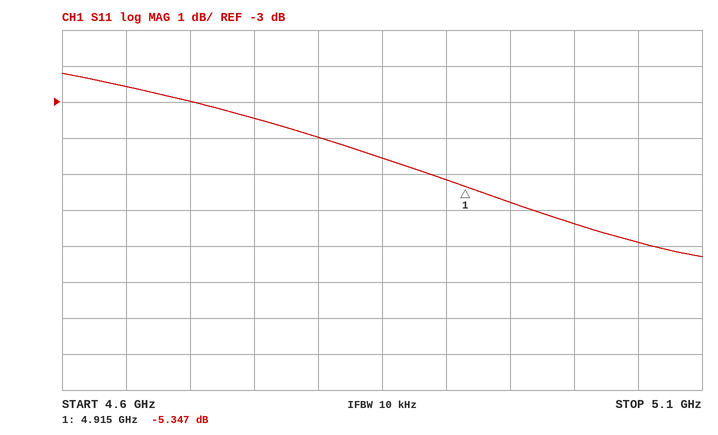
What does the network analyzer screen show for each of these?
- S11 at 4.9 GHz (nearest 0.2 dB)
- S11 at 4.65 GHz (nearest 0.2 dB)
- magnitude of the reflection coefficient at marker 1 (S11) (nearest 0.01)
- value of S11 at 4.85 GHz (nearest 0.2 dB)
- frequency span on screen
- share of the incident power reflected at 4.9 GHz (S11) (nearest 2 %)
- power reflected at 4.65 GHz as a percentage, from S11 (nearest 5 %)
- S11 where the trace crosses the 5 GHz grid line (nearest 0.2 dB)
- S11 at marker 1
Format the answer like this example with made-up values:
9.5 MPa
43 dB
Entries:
-5.2 dB
-2.6 dB
0.54
-4.6 dB
500 MHz
30 %
55 %
-6.4 dB
-5.347 dB
